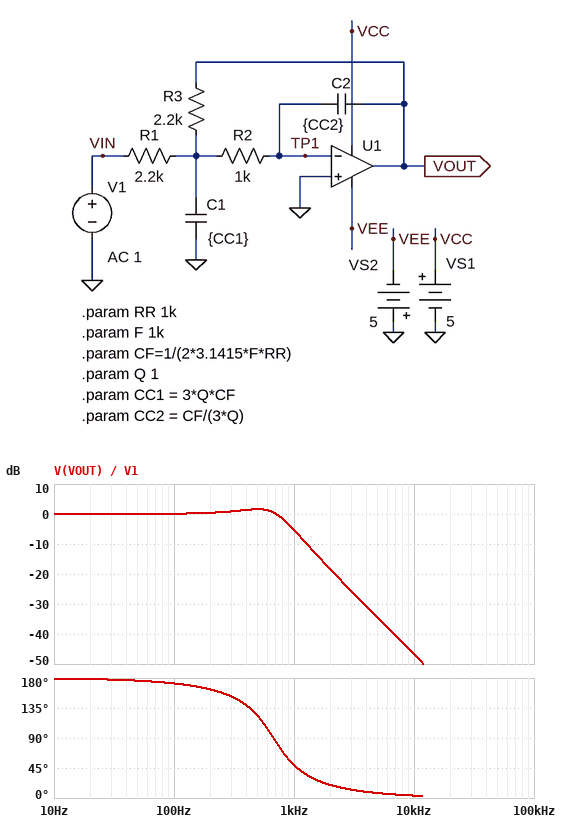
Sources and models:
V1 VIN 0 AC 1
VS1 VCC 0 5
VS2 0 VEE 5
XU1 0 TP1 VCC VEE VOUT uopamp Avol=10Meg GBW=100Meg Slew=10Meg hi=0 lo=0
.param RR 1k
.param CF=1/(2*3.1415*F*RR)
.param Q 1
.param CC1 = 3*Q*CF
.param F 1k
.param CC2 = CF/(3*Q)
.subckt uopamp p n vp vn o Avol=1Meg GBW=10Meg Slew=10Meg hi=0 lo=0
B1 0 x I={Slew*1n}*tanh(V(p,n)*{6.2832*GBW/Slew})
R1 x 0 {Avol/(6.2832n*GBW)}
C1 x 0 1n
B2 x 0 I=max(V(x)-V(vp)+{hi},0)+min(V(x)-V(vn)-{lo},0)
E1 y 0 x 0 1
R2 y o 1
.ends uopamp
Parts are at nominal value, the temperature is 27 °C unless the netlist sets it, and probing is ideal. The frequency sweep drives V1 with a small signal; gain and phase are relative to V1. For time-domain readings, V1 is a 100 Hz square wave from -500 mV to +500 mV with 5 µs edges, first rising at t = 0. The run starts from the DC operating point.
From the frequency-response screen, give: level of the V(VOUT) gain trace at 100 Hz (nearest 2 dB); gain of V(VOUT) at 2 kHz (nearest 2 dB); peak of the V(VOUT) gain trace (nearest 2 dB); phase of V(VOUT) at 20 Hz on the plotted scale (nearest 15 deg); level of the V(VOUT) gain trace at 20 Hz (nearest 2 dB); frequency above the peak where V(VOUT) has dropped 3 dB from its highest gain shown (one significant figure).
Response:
0 dB
-18 dB
2 dB
180 deg
0 dB
800 Hz
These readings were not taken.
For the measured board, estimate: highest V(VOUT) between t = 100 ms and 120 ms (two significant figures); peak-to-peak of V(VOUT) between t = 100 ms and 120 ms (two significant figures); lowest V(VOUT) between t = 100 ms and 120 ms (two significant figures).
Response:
690 mV
1.4 V
-690 mV
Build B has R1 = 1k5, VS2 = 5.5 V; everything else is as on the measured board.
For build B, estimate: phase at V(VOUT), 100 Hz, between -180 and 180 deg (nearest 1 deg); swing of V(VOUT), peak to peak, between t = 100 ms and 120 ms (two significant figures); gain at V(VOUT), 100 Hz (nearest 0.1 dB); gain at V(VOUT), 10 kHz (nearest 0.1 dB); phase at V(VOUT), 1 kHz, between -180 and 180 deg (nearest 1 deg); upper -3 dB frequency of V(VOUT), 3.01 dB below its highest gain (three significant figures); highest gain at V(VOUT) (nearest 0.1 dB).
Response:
171 deg
1.9 V
3.4 dB
-43.5 dB
52 deg
781 Hz
4.3 dB
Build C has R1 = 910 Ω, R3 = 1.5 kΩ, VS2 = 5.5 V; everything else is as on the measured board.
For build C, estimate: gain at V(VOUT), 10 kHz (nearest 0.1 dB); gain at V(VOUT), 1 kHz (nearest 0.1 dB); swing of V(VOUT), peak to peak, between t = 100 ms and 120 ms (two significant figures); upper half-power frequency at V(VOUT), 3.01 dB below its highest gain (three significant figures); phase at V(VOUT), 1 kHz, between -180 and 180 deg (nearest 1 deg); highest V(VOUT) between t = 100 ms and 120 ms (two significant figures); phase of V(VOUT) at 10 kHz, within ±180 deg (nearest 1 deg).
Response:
-39.2 dB
1.0 dB
2.0 V
929 Hz
70 deg
1.0 V
5 deg
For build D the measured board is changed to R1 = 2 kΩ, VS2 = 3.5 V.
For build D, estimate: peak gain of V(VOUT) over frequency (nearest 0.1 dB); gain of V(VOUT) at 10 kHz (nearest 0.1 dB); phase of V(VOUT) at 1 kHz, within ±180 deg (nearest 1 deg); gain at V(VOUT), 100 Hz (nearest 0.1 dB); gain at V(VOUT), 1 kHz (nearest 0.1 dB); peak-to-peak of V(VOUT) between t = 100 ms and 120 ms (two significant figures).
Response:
2.3 dB
-46.0 dB
50 deg
0.9 dB
-4.6 dB
1.5 V
